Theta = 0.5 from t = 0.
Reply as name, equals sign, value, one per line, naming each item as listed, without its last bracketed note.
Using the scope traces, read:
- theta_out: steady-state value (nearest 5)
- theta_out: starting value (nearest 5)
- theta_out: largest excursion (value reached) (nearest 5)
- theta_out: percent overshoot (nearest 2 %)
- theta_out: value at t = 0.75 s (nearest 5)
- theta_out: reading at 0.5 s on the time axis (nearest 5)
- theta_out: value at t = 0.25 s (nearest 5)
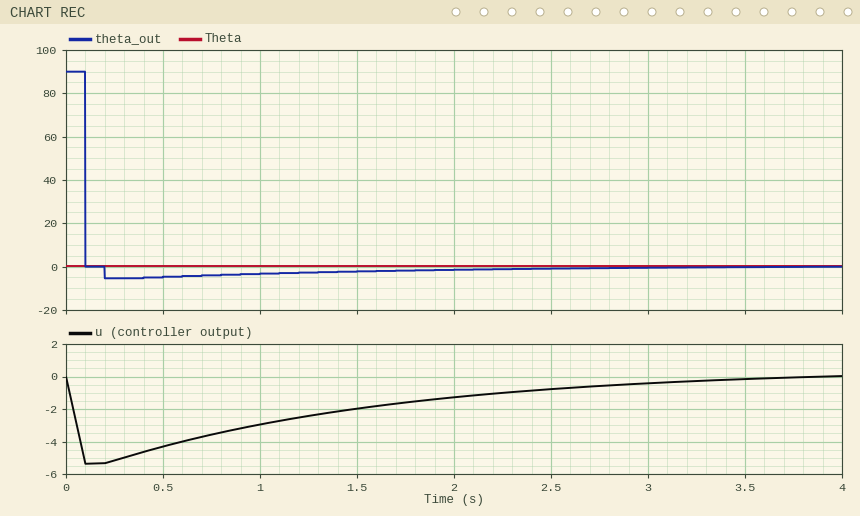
theta_out: steady-state value = 0
theta_out: starting value = 90
theta_out: largest excursion (value reached) = -5
theta_out: percent overshoot = 6 %
theta_out: value at t = 0.75 s = -5
theta_out: reading at 0.5 s on the time axis = -5
theta_out: value at t = 0.25 s = -5
